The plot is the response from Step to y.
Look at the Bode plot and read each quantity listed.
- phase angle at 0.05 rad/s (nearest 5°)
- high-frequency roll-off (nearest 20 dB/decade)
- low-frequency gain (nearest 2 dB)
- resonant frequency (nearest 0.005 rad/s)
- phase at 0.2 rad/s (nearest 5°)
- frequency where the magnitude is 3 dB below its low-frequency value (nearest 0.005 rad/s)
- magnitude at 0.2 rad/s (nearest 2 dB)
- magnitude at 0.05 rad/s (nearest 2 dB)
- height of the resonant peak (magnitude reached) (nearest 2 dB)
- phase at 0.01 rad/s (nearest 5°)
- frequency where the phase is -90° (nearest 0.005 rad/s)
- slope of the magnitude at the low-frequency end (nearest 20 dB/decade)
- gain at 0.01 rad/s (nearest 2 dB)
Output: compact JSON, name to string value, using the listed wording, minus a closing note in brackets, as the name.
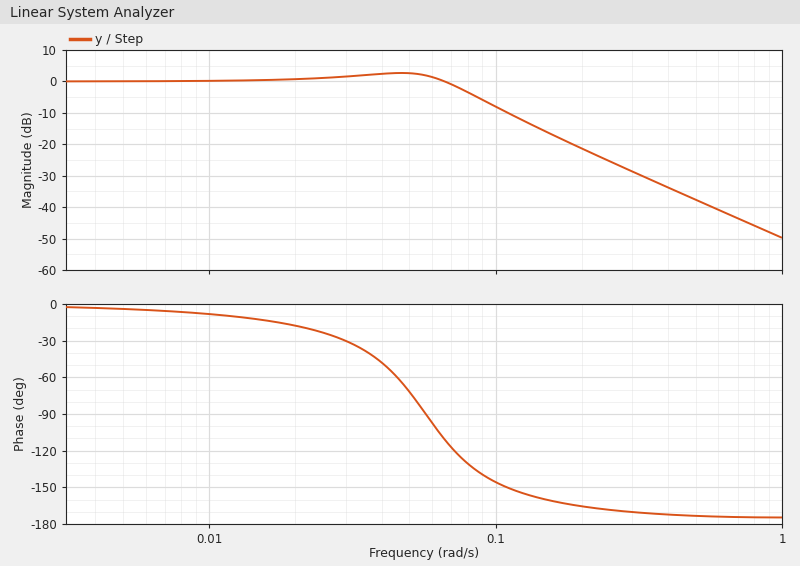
{"phase angle at 0.05 rad/s": "-70°", "high-frequency roll-off": "-40 dB/decade", "low-frequency gain": "0 dB", "resonant frequency": "0.045 rad/s", "phase at 0.2 rad/s": "-165°", "frequency where the magnitude is 3 dB below its low-frequency value": "0.080 rad/s", "magnitude at 0.2 rad/s": "-22 dB", "magnitude at 0.05 rad/s": "2 dB", "height of the resonant peak (magnitude reached)": "2 dB", "phase at 0.01 rad/s": "-10°", "frequency where the phase is -90°": "0.055 rad/s", "slope of the magnitude at the low-frequency end": "0 dB/decade", "gain at 0.01 rad/s": "0 dB"}
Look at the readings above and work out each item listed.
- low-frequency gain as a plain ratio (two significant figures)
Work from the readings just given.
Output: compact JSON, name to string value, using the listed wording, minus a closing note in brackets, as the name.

{"low-frequency gain as a plain ratio": "1.0"}
